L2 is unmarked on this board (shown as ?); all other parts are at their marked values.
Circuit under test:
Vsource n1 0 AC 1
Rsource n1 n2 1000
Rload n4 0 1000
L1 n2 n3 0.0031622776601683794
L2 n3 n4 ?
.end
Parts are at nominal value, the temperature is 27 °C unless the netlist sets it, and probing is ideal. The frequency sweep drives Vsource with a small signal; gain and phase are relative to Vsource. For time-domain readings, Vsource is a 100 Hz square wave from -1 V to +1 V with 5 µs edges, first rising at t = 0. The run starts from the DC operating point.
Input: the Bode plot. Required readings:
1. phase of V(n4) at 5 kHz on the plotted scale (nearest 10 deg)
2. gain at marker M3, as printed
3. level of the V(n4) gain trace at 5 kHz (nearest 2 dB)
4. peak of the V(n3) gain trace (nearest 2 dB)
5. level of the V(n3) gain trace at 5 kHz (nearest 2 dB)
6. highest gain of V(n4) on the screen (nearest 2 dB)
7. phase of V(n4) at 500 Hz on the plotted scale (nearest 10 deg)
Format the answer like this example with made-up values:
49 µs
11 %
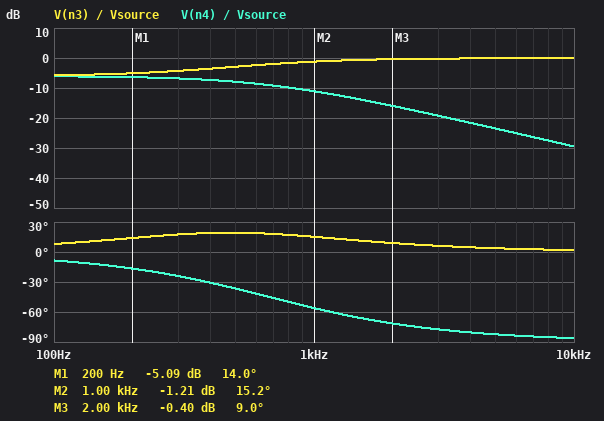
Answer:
-80 deg
-0.40 dB
-24 dB
0 dB
0 dB
-6 dB
-40 deg
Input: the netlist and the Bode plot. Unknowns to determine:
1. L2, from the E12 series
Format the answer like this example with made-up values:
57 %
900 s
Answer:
470 mH
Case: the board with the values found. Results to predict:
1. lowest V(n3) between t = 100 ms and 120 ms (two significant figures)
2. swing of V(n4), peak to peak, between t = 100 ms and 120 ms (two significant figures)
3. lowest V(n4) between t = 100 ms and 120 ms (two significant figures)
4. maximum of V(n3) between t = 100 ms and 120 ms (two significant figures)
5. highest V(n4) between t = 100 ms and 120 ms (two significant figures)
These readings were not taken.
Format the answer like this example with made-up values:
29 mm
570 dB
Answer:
-1.5 V
1.0 V
-500 mV
1.5 V
500 mV
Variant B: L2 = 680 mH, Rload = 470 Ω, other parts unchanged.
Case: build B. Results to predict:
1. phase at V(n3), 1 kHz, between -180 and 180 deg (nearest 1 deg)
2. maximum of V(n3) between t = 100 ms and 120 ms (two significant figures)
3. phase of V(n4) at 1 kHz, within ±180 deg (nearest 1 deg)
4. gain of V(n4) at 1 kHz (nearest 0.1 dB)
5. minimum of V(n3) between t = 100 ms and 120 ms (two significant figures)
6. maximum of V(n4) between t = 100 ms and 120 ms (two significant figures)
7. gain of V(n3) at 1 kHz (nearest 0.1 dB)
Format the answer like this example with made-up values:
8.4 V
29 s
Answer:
13 deg
1.7 V
-71 deg
-19.7 dB
-1.7 V
320 mV
-0.5 dB
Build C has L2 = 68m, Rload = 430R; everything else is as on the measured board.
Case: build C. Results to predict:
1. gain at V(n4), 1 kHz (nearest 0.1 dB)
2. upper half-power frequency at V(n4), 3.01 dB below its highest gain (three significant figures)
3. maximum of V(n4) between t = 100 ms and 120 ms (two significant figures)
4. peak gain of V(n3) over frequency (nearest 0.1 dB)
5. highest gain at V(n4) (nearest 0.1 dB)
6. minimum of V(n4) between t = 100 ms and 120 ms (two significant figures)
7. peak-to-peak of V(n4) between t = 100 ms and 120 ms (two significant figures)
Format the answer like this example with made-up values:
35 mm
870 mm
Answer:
-10.8 dB
3.20 kHz
300 mV
-0.4 dB
-10.4 dB
-300 mV
600 mV
